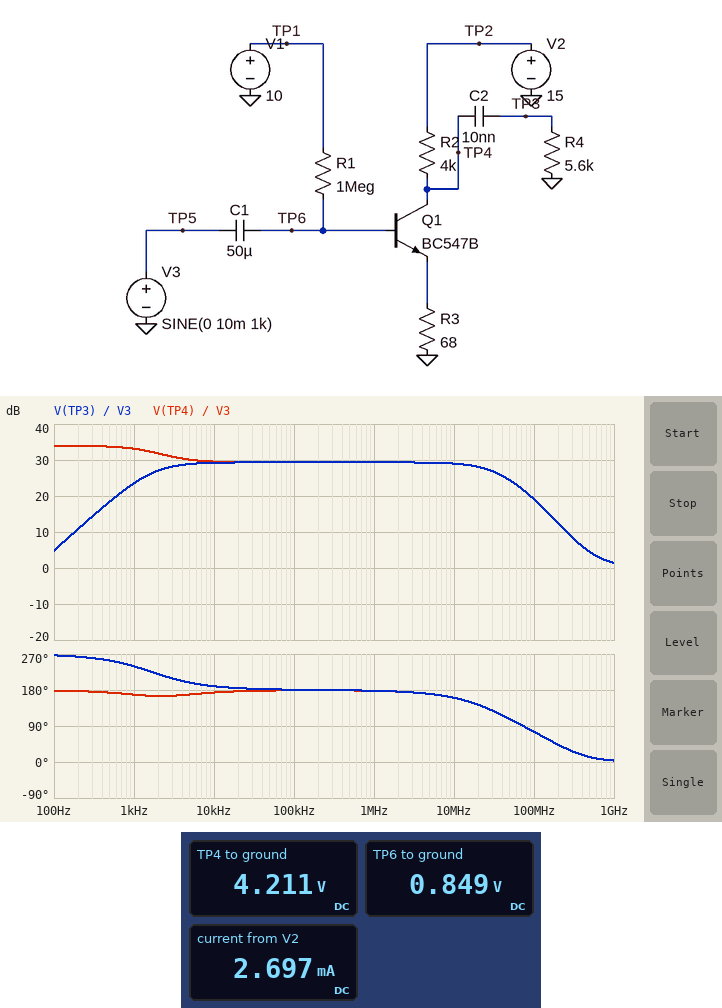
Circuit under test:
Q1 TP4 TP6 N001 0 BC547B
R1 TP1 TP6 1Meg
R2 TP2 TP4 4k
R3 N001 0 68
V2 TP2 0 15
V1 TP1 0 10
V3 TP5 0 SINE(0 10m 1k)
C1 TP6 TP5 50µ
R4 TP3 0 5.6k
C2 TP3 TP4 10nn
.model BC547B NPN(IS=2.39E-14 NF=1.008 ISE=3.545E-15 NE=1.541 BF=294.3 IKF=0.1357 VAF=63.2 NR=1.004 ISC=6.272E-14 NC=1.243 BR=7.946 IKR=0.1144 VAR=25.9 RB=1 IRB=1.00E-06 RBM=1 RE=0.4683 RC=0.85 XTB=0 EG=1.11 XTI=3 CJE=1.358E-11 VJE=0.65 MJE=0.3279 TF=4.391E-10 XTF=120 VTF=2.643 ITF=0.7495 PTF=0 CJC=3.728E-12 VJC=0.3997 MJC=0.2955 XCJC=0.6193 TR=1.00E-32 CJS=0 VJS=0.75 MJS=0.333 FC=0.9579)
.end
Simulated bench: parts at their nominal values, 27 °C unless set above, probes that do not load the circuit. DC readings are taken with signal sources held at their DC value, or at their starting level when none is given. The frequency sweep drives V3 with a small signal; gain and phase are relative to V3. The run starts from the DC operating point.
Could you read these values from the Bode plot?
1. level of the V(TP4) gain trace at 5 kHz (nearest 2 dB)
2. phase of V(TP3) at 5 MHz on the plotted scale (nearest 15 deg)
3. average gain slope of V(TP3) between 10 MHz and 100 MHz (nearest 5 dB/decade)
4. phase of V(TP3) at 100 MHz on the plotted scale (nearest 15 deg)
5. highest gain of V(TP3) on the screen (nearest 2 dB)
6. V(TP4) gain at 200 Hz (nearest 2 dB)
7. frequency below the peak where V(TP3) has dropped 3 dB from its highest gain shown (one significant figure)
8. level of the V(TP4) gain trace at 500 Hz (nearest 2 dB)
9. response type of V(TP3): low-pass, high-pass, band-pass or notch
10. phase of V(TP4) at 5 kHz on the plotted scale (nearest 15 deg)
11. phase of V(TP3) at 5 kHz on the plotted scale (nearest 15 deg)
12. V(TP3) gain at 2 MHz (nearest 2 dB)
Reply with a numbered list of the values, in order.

1. 30 dB
2. 165 deg
3. -10 dB/decade
4. 75 deg
5. 30 dB
6. 34 dB
7. 2 kHz
8. 34 dB
9. band-pass
10. 165 deg
11. 195 deg
12. 30 dB
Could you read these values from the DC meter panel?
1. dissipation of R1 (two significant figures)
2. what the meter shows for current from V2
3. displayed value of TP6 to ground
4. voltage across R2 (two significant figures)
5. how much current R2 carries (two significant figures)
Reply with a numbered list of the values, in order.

1. 84 µW
2. 2.697 mA
3. 0.849 V
4. 11 V
5. 2.7 mA
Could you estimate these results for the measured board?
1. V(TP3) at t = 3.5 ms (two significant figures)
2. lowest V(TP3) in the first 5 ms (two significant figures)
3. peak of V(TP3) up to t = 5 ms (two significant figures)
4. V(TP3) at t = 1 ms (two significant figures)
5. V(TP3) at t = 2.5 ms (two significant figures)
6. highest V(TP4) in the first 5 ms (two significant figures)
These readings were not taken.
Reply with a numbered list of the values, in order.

1. 130 mV
2. -150 mV
3. 150 mV
4. -130 mV
5. 130 mV
6. 4.7 V
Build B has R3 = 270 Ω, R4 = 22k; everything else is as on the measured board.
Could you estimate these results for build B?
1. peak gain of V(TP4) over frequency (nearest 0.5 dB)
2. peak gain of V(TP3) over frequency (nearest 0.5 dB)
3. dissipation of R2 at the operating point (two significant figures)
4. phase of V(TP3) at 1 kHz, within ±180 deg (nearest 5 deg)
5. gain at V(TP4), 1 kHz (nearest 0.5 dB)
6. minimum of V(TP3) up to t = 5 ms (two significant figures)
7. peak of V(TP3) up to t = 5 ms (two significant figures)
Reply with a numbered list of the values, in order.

1. 23.0 dB
2. 21.5 dB
3. 26 mW
4. -150 deg
5. 22.0 dB
6. -100 mV
7. 110 mV
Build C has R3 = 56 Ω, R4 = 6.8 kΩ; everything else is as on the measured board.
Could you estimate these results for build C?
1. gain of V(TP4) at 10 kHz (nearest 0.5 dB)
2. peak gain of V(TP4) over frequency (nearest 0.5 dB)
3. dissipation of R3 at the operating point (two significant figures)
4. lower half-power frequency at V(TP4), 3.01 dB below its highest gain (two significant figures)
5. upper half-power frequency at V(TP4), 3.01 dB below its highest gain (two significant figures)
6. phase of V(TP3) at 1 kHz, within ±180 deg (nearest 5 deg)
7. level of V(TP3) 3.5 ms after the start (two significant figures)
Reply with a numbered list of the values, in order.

1. 31.5 dB
2. 35.5 dB
3. 410 µW
4. 190 mHz
5. 3.4 kHz
6. -125 deg
7. 170 mV
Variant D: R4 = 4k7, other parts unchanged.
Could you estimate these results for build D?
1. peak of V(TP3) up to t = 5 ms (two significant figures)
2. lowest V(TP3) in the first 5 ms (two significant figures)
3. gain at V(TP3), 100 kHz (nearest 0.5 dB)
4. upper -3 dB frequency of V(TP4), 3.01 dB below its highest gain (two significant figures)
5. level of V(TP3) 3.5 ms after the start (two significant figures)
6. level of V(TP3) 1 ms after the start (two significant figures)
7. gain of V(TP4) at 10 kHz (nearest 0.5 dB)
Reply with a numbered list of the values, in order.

1. 130 mV
2. -130 mV
3. 28.5 dB
4. 2.9 kHz
5. 110 mV
6. -110 mV
7. 29.0 dB
